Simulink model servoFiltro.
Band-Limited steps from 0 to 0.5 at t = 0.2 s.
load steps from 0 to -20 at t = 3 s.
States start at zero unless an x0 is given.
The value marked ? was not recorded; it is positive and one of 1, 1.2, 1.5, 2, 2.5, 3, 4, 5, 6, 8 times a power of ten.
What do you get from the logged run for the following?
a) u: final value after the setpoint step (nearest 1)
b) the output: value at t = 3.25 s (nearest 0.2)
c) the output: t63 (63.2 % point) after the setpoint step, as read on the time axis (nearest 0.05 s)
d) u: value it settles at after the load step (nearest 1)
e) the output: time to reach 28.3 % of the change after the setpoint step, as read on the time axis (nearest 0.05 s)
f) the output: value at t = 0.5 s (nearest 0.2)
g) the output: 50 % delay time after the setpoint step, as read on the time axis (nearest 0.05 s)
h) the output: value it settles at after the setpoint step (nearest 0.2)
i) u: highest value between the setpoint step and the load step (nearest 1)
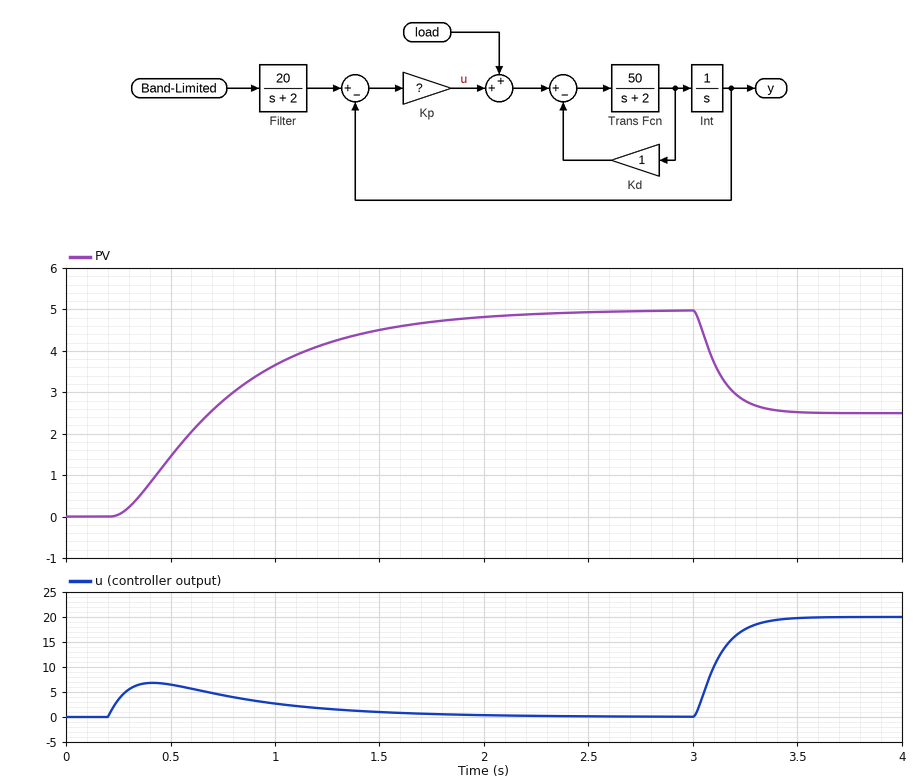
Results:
0
2.8
0.85 s
20
0.50 s
1.4
0.70 s
5.0
7
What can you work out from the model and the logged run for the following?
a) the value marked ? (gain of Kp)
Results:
8
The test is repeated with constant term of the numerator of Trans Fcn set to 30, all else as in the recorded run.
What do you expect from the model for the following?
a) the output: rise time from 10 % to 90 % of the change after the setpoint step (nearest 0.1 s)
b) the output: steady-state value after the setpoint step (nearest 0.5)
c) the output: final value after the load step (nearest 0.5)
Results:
1.1 s
5.0
2.5
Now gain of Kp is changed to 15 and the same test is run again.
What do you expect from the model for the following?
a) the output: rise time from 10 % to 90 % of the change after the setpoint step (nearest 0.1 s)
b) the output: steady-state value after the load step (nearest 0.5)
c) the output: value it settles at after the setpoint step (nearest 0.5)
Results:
1.1 s
3.5
5.0
